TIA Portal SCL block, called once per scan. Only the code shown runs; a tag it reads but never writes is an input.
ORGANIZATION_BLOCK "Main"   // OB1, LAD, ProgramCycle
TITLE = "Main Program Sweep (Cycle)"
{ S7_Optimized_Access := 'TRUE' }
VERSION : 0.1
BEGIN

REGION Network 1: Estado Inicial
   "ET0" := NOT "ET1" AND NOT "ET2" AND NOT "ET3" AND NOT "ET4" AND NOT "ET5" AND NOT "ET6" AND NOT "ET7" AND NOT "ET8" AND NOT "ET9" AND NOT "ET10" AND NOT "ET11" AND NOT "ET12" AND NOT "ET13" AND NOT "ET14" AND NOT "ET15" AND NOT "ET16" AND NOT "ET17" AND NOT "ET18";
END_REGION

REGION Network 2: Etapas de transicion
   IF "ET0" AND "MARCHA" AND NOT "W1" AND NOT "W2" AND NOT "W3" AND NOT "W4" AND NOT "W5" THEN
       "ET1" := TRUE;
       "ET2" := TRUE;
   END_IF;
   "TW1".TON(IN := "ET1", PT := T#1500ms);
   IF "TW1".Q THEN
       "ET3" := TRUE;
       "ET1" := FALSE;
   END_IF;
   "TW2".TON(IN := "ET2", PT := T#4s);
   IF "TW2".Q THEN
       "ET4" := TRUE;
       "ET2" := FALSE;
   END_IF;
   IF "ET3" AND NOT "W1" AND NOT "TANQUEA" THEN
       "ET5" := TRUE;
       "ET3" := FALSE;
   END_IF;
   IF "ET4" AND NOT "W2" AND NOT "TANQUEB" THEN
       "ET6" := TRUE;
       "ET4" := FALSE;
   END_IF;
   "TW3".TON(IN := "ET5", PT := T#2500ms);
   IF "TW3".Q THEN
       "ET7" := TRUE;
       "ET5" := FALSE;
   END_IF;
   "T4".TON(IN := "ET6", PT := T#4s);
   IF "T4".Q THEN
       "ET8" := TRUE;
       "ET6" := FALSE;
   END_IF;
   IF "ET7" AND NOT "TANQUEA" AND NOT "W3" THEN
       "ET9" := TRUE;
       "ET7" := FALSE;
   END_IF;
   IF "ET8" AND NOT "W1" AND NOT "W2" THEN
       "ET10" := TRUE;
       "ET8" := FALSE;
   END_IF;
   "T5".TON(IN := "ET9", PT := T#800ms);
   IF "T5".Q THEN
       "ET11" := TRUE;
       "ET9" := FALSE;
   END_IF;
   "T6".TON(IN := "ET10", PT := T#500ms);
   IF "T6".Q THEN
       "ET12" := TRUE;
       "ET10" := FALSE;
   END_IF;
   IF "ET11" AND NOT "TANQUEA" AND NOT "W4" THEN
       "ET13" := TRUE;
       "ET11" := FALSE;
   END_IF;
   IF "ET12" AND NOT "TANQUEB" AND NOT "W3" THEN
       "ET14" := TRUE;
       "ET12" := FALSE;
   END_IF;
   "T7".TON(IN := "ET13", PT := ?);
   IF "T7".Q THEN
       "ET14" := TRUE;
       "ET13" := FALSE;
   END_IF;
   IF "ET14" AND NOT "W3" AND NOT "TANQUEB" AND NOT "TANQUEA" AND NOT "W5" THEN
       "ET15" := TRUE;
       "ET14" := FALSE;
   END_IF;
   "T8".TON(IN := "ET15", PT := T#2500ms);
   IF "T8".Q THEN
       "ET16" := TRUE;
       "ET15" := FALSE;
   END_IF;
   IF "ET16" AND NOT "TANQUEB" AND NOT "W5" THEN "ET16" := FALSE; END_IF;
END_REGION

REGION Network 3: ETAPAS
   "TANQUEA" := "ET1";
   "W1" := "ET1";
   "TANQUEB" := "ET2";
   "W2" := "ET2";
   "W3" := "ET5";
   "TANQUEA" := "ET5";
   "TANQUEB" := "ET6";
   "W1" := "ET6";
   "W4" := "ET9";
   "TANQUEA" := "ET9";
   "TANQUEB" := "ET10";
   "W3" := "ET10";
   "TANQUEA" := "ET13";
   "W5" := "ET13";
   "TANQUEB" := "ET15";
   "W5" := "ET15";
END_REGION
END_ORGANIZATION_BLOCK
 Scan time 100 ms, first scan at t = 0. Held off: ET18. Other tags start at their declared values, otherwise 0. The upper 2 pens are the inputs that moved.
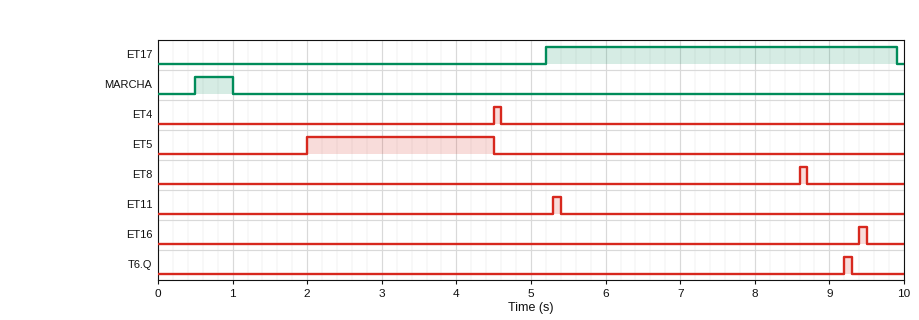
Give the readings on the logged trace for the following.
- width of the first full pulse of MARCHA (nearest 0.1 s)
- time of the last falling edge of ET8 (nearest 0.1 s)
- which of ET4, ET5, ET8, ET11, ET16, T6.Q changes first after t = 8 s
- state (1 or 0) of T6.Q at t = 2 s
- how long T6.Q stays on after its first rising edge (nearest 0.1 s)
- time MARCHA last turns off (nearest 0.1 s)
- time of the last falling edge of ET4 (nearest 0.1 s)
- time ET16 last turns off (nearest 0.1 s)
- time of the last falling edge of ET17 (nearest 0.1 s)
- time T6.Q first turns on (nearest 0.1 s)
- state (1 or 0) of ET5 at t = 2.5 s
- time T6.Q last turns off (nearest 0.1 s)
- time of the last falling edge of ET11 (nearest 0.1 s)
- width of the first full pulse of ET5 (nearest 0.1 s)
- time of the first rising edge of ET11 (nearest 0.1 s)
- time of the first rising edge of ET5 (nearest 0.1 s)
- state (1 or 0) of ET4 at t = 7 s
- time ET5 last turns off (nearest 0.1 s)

0.5 s
8.7 s
ET8
0
0.1 s
1.0 s
4.6 s
9.5 s
9.9 s
9.2 s
1
9.3 s
5.4 s
2.5 s
5.3 s
2.0 s
0
4.5 s
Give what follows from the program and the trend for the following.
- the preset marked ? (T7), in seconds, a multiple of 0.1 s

1.4 s
